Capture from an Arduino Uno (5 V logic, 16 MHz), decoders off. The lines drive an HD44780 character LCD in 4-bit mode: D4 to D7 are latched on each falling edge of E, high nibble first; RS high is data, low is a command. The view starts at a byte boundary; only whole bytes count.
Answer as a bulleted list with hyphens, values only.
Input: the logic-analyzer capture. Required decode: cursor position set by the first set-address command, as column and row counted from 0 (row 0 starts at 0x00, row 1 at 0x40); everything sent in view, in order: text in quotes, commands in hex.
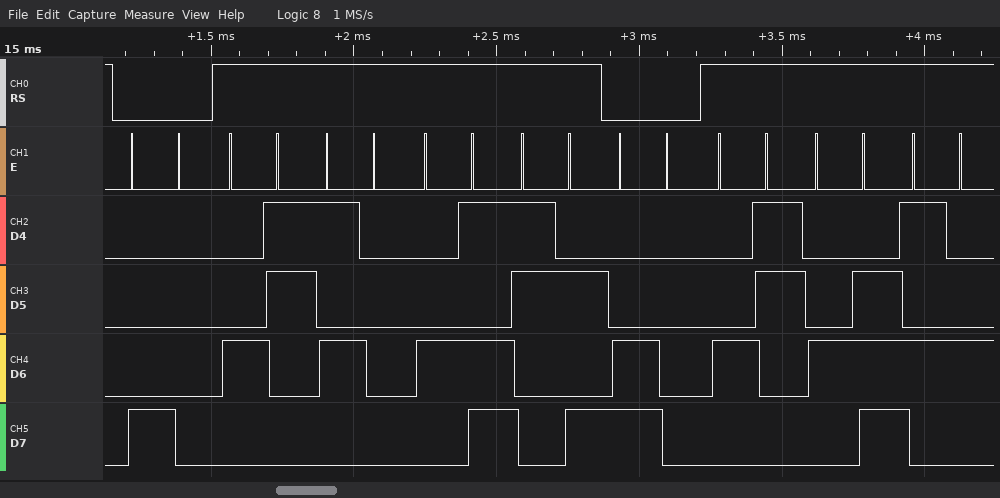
- column 0, row 0
- 0x80 "CPM:" 0xC0 "CNT"
